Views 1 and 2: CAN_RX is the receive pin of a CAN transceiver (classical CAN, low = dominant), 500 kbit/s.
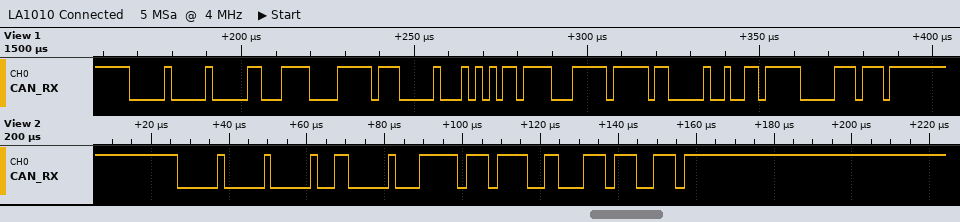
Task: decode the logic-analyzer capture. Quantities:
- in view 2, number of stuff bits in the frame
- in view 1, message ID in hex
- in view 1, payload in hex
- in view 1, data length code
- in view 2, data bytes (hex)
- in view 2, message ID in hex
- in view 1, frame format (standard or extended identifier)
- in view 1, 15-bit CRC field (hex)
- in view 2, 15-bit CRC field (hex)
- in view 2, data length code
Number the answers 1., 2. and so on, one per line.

1. 5
2. 0x000
3. F0 FF 00 AB 78 FF F0 13
4. 8
5. 00 FF 79
6. 0x000
7. standard
8. 0x3E1B
9. 0x4773
10. 3
